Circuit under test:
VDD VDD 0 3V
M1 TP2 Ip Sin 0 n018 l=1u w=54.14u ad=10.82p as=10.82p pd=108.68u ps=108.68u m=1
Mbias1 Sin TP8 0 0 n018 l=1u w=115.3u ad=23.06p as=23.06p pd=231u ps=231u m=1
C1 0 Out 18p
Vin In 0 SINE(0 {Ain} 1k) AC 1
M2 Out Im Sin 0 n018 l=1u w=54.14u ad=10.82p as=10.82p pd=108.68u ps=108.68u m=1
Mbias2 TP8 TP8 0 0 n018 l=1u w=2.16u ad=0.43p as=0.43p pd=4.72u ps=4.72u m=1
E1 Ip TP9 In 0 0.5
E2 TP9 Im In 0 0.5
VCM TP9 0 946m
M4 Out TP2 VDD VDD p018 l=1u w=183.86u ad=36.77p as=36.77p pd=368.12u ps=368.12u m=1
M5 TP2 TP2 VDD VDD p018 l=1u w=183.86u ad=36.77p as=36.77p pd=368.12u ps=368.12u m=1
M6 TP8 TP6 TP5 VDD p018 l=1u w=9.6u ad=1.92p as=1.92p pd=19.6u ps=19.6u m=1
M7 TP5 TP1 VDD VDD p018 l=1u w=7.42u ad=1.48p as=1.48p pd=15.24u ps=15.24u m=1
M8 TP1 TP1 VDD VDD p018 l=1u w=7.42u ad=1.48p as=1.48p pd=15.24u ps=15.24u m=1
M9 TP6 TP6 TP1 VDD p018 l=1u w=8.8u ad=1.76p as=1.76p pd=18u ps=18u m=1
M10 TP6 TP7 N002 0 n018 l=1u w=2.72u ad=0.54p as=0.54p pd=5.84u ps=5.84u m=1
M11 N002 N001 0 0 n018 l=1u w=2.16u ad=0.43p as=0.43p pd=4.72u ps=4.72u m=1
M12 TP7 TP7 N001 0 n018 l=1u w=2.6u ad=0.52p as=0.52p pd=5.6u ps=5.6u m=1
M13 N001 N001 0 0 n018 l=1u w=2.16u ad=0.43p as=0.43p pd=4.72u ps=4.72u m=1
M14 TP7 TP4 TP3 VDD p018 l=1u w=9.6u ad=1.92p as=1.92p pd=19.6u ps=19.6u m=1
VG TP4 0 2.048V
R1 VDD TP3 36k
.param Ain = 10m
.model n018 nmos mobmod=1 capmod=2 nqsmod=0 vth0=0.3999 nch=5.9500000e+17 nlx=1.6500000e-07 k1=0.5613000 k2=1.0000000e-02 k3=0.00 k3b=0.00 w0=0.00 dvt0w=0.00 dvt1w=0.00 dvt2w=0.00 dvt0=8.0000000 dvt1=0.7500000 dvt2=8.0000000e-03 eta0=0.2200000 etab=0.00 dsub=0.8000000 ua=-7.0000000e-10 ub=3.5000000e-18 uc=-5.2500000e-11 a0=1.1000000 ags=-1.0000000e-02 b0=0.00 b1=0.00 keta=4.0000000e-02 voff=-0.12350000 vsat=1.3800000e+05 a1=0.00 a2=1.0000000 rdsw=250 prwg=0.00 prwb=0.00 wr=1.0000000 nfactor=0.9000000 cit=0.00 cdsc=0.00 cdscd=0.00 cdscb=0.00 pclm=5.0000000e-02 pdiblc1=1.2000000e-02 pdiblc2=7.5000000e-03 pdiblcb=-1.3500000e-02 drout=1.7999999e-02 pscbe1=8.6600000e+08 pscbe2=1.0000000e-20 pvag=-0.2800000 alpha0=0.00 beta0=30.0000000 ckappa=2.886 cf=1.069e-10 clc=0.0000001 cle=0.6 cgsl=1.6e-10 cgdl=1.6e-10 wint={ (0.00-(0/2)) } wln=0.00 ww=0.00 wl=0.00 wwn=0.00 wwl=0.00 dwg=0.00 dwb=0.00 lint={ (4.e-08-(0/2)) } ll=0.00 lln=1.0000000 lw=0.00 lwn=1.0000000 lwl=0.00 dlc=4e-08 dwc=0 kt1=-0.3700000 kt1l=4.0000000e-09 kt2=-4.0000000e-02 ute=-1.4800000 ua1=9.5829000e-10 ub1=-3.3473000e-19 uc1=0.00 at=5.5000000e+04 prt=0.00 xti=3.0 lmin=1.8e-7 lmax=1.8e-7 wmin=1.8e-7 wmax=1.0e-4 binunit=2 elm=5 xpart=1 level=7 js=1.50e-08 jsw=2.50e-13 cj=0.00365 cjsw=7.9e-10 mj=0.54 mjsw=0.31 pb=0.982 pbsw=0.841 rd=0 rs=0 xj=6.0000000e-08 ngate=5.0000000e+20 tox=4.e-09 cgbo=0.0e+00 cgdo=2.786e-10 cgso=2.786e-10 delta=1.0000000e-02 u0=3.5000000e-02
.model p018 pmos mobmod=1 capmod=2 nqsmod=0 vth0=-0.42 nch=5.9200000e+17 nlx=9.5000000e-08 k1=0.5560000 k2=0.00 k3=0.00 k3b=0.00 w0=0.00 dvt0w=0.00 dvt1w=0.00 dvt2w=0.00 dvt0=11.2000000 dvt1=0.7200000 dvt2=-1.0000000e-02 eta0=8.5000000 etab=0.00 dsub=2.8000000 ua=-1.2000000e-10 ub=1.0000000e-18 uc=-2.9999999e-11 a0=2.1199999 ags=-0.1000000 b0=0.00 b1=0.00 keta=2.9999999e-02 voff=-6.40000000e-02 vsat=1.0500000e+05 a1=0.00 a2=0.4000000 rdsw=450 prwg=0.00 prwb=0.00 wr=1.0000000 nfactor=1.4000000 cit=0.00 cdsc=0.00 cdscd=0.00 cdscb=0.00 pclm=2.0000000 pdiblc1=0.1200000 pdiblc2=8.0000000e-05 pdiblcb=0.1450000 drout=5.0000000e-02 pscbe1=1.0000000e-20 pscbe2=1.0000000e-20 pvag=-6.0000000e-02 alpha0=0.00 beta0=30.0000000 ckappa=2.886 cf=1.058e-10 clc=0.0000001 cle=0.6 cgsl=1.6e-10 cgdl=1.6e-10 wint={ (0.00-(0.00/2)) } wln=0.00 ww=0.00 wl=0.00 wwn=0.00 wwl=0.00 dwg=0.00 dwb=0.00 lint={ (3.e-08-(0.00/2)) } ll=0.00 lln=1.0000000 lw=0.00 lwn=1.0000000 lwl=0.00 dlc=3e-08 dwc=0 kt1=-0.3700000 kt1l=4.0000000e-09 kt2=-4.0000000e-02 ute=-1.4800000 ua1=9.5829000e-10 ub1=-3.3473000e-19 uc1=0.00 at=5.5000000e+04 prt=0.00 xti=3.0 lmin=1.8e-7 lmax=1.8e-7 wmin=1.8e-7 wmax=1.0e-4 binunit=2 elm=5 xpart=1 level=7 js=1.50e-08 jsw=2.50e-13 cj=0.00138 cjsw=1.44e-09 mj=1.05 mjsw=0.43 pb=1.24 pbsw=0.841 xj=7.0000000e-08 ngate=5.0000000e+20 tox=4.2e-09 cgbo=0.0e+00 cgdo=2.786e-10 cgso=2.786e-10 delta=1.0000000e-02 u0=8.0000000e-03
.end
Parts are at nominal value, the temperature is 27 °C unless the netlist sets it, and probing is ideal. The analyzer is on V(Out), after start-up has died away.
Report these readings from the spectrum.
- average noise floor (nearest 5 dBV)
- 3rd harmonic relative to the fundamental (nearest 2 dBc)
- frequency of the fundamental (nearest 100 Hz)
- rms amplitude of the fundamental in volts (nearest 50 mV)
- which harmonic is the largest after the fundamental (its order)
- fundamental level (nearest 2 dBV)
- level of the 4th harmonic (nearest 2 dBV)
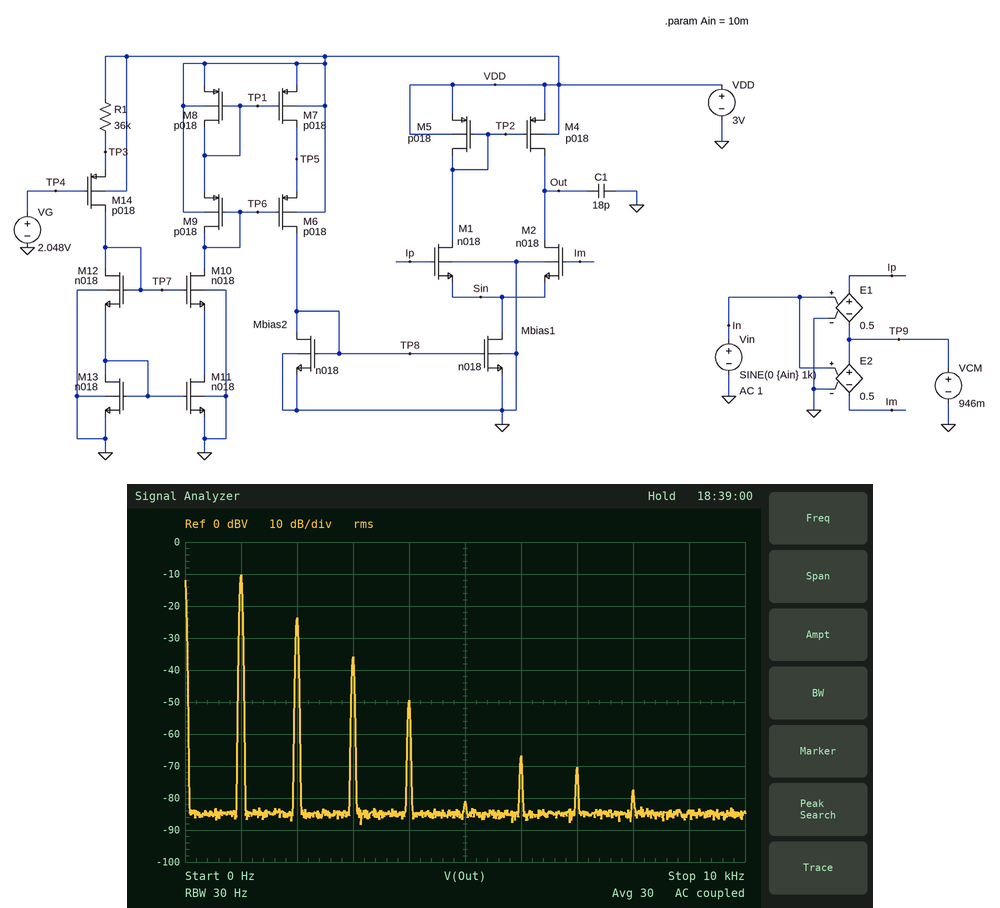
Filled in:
-85 dBV
-26 dBc
1.0 kHz
300 mV
2
-10 dBV
-50 dBV
